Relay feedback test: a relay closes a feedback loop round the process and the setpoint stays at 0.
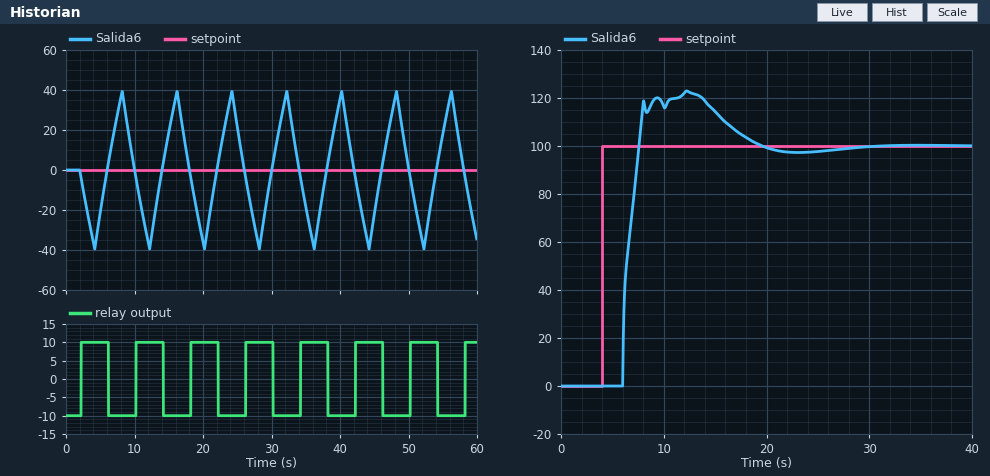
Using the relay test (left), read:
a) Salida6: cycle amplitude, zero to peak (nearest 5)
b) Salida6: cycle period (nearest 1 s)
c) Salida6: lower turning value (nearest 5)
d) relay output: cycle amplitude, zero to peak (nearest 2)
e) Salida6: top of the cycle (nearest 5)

40
8 s
-40
10
40
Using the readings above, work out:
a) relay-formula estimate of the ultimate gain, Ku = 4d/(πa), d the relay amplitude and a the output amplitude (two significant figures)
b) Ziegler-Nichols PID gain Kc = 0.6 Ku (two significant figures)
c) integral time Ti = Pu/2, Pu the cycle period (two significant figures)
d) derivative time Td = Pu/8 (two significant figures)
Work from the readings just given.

0.32
0.19
4.0 s
1.0 s
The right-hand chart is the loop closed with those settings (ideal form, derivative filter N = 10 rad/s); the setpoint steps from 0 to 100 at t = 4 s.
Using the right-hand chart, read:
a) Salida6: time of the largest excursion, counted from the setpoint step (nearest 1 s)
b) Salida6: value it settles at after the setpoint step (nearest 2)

8 s
100
